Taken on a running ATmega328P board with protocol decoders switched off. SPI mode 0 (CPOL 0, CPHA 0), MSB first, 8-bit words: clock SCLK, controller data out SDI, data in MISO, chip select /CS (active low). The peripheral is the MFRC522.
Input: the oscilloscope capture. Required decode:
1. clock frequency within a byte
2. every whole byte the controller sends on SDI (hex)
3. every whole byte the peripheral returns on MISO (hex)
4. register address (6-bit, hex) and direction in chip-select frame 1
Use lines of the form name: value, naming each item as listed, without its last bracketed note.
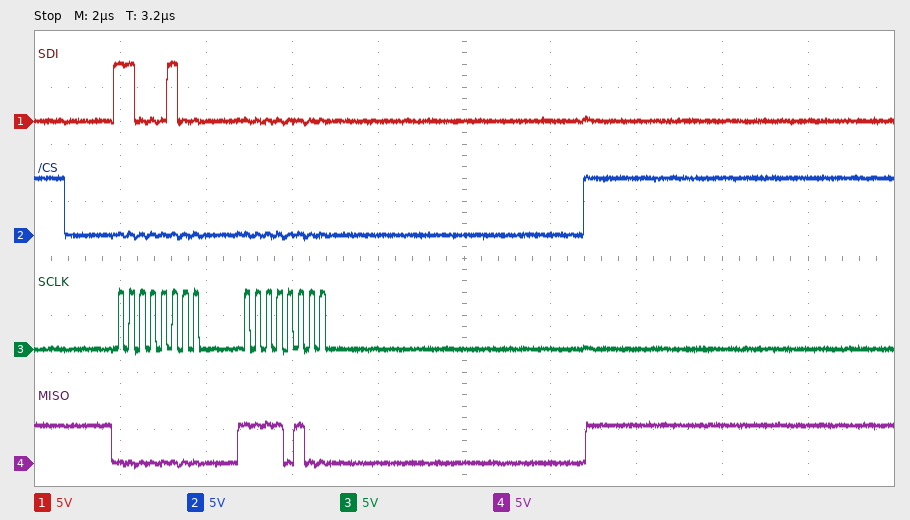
clock frequency within a byte: 4 MHz
every whole byte the controller sends on SDI: 0xC4 0x00
every whole byte the peripheral returns on MISO: 0x00 0xF4
register address (6-bit, hex) and direction in chip-select frame 1: 0x22 read
